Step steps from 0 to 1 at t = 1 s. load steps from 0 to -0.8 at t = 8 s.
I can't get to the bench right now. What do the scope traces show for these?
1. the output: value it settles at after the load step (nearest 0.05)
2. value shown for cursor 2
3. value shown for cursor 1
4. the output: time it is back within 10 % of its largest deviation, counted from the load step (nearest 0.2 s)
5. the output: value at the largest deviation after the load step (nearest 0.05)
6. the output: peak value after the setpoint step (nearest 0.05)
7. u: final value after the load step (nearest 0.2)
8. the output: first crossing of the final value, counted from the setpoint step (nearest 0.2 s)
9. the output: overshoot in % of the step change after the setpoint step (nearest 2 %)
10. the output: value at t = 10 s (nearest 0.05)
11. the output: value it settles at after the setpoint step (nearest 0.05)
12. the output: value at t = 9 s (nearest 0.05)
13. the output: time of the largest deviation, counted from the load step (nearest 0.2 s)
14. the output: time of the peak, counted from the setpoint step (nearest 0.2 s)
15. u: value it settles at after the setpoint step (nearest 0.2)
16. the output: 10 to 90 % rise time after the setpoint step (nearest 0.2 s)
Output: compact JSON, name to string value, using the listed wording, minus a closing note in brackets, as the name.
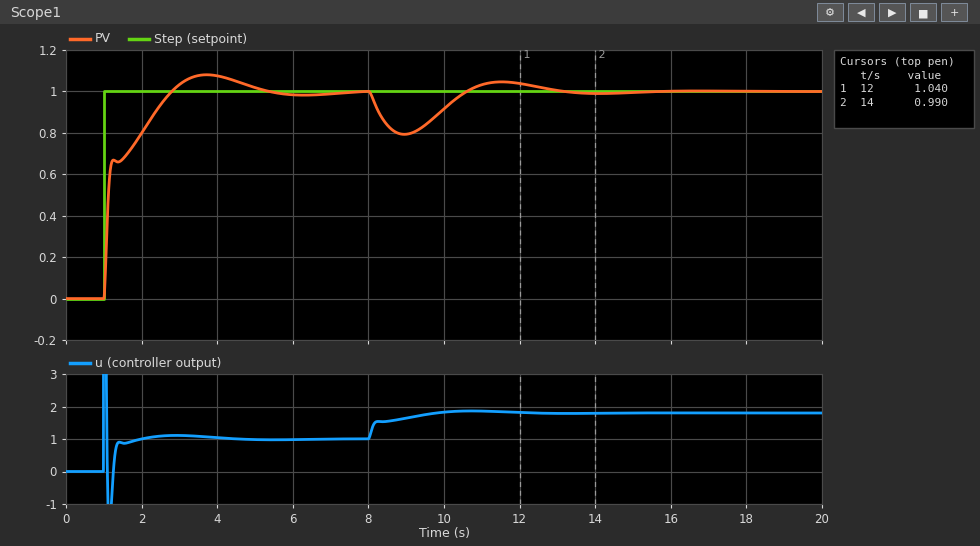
{"the output: value it settles at after the load step": "1.00", "value shown for cursor 2": "0.990", "value shown for cursor 1": "1.040", "the output: time it is back within 10 % of its largest deviation, counted from the load step": "4.6 s", "the output: value at the largest deviation after the load step": "0.80", "the output: peak value after the setpoint step": "1.10", "u: final value after the load step": "1.8", "the output: first crossing of the final value, counted from the setpoint step": "1.8 s", "the output: overshoot in % of the step change after the setpoint step": "8 %", "the output: value at t = 10 s": "0.90", "the output: value it settles at after the setpoint step": "1.00", "the output: value at t = 9 s": "0.80", "the output: time of the largest deviation, counted from the load step": "1.0 s", "the output: time of the peak, counted from the setpoint step": "2.8 s", "u: value it settles at after the setpoint step": "1.0", "the output: 10 to 90 % rise time after the setpoint step": "1.4 s"}
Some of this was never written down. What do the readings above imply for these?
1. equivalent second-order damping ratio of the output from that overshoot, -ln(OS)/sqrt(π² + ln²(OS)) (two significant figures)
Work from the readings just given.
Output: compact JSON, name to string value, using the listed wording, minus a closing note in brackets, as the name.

{"equivalent second-order damping ratio of the output from that overshoot, -ln(OS)/sqrt(π² + ln²(OS))": "0.63"}
